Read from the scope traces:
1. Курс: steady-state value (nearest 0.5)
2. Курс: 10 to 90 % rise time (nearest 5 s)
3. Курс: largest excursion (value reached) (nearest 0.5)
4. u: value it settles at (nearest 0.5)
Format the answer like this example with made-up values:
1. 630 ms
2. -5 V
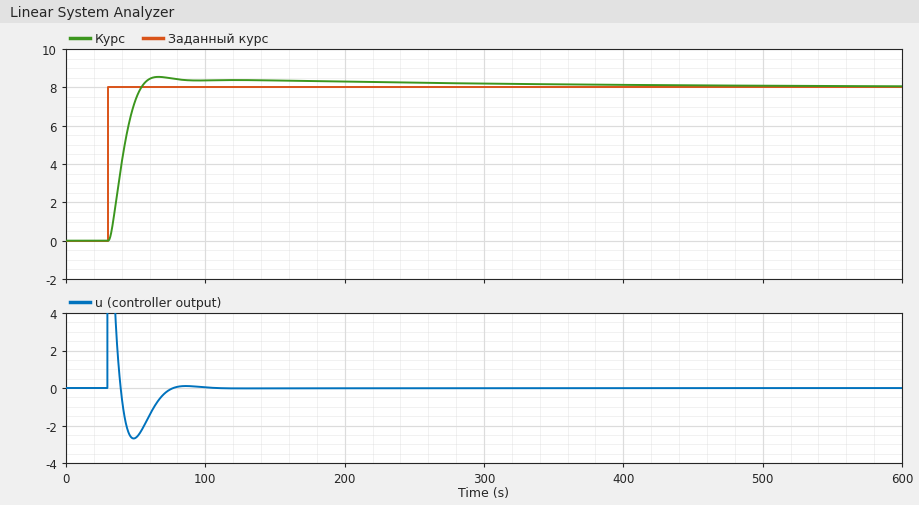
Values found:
1. 8.0
2. 15 s
3. 8.5
4. 0.0
